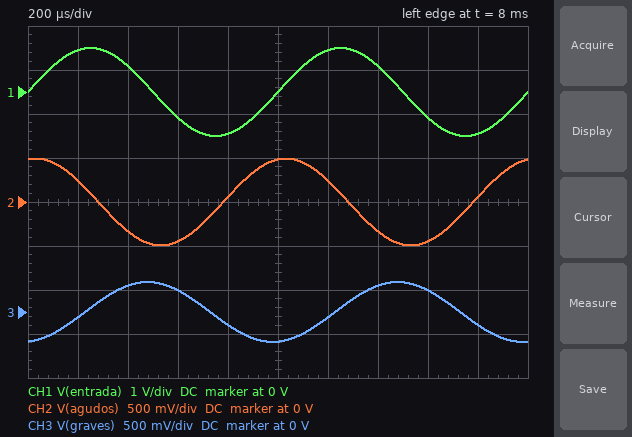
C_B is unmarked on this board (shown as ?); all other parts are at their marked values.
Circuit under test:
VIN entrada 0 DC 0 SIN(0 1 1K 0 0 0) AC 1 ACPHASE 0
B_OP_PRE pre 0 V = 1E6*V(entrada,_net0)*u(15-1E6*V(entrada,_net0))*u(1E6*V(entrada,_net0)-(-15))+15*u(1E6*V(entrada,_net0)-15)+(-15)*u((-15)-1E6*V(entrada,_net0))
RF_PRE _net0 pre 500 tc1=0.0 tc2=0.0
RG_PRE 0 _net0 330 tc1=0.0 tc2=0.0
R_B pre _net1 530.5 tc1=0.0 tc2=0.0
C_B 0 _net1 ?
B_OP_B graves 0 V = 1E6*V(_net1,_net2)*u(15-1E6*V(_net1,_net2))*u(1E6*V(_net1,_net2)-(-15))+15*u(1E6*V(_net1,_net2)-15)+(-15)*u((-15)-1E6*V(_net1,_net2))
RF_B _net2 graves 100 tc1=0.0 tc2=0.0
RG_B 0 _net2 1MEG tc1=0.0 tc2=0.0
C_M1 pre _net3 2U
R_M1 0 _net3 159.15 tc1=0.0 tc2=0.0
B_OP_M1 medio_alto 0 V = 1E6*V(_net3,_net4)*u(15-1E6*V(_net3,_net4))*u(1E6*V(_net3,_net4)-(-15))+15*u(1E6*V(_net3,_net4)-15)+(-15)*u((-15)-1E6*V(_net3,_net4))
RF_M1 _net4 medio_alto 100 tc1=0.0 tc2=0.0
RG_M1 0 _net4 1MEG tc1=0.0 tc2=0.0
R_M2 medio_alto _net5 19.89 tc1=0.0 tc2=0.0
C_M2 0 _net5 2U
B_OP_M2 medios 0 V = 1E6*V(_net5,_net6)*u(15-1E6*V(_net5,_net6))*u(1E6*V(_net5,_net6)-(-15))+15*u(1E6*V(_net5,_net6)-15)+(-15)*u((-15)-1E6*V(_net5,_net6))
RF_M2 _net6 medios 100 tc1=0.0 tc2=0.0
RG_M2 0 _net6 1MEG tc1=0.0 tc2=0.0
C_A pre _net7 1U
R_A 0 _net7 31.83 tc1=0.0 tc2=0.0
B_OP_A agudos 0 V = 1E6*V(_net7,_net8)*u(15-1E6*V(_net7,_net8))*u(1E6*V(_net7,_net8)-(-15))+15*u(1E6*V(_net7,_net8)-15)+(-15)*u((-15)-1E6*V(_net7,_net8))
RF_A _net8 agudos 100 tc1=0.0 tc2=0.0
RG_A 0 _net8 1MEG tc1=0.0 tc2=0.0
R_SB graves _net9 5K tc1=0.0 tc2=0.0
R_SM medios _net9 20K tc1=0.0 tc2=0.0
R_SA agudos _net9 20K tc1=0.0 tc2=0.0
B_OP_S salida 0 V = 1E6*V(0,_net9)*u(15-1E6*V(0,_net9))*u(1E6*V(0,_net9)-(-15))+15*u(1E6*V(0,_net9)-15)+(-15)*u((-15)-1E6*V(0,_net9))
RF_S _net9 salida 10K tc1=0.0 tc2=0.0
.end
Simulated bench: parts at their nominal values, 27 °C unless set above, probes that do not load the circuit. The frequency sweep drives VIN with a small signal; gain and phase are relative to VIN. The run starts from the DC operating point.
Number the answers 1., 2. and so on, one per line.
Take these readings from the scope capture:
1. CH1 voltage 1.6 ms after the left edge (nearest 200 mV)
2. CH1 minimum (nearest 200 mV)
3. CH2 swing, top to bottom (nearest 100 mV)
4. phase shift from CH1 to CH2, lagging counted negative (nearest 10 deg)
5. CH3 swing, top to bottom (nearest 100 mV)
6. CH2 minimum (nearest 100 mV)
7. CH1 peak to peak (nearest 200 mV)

1. -600 mV
2. -1.0 V
3. 1.0 V
4. 80 deg
5. 700 mV
6. -500 mV
7. 2.0 V
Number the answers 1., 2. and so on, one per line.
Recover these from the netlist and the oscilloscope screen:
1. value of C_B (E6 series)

1. 2.2 µF
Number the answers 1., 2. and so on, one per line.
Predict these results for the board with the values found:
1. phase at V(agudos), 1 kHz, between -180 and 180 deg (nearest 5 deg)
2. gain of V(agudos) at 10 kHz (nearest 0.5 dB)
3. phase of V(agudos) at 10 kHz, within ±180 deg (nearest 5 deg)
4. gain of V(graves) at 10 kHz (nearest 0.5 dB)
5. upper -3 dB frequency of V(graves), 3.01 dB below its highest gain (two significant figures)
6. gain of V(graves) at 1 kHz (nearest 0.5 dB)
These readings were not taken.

1. 80 deg
2. 7.0 dB
3. 25 deg
4. -29.5 dB
5. 140 Hz
6. -9.5 dB
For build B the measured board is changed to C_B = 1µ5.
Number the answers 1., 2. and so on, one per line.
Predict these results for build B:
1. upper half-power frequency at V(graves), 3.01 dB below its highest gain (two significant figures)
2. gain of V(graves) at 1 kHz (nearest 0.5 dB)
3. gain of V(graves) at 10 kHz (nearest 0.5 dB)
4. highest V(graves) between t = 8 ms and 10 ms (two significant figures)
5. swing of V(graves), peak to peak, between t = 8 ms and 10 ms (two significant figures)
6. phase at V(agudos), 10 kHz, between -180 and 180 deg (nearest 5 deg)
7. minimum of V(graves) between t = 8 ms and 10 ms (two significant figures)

1. 200 Hz
2. -6.0 dB
3. -26.0 dB
4. 490 mV
5. 990 mV
6. 25 deg
7. -490 mV
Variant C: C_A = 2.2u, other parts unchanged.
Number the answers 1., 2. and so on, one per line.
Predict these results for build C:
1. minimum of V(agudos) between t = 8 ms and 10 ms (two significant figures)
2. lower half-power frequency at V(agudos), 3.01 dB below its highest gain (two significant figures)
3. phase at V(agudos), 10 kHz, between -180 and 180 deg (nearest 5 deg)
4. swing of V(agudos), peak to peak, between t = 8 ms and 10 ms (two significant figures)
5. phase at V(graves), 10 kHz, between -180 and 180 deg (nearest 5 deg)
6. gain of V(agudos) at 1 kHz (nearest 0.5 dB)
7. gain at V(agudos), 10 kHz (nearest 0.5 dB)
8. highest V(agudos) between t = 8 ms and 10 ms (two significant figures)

1. -1.0 V
2. 2.3 kHz
3. 15 deg
4. 2.0 V
5. -90 deg
6. 0 dB
7. 8.0 dB
8. 1.0 V
